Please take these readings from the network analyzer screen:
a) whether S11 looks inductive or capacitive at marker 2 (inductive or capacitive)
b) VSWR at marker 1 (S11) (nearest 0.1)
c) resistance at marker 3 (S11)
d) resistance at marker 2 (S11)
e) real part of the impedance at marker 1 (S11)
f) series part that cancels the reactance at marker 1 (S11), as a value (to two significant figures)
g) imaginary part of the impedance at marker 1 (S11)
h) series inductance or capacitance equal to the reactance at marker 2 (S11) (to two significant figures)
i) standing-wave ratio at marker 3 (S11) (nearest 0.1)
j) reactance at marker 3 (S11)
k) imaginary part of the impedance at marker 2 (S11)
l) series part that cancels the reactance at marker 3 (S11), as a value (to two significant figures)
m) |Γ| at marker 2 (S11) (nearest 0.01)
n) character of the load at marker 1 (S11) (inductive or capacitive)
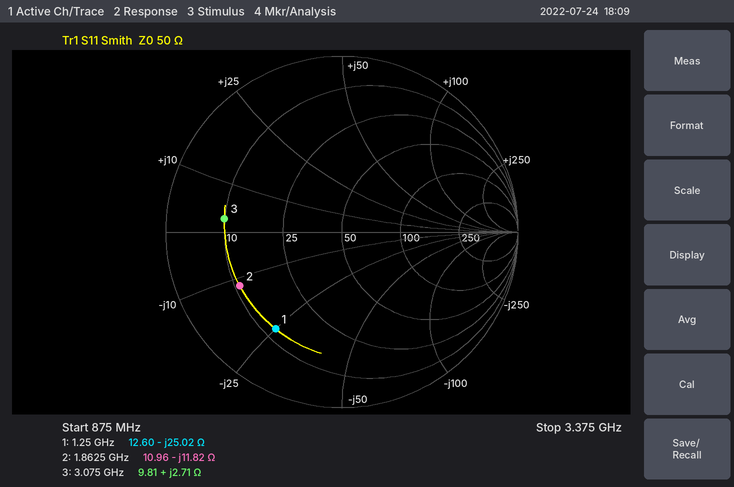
capacitive
5.0
9.81 Ω
10.96 Ω
12.60 Ω
3.2 nH
-25.02 Ω
7.2 pF
5.1
+2.71 Ω
-11.82 Ω
19 pF
0.66
capacitive
